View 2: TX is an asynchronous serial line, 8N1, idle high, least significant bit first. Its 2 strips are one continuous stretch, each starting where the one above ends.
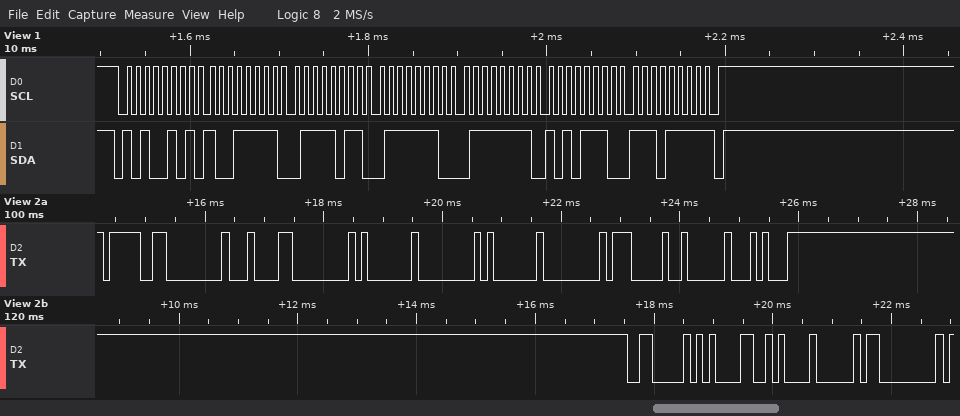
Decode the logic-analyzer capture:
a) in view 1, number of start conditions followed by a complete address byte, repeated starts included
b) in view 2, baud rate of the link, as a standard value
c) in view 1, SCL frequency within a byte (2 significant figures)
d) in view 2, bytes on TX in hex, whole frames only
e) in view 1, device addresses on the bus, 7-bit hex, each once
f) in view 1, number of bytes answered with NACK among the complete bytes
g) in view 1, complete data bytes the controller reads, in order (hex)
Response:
1
9600 baud
100 kHz
0x9F 0x00 0x84 0x00 0x01 0x00 0x01 0x00 0x07 0x02 0x14 0x06 0x85 0x0A 0xA0 0x00
0x52
1
9F 7B 7E 7F AE EF
